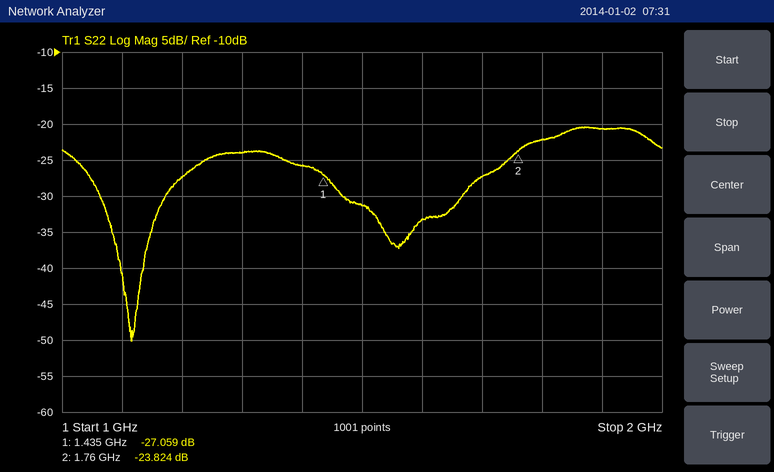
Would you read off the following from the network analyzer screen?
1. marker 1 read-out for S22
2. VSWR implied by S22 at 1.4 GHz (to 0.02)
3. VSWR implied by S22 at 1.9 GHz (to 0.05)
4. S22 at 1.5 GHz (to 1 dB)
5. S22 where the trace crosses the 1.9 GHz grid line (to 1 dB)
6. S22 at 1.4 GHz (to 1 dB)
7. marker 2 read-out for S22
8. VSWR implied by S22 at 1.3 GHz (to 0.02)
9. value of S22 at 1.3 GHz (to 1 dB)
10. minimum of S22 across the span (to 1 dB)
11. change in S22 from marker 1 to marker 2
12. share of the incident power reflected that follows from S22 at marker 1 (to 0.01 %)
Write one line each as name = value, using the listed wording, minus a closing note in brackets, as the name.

marker 1 read-out for S22 = -27.059 dB
VSWR implied by S22 at 1.4 GHz = 1.10
VSWR implied by S22 at 1.9 GHz = 1.20
S22 at 1.5 GHz = -31 dB
S22 where the trace crosses the 1.9 GHz grid line = -21 dB
S22 at 1.4 GHz = -26 dB
marker 2 read-out for S22 = -23.824 dB
VSWR implied by S22 at 1.3 GHz = 1.14
value of S22 at 1.3 GHz = -24 dB
minimum of S22 across the span = -50 dB
change in S22 from marker 1 to marker 2 = 3.235 dB
share of the incident power reflected that follows from S22 at marker 1 = 0.20 %
